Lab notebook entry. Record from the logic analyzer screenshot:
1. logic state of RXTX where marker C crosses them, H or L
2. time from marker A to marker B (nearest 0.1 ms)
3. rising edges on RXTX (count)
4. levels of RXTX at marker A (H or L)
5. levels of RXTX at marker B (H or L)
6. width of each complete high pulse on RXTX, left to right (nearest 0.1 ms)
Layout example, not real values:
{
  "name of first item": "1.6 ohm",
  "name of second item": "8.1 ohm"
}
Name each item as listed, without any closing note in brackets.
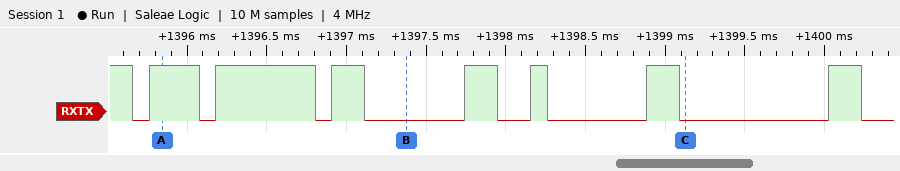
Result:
{
  "logic state of RXTX where marker C crosses them, H or L": "RXTX=L",
  "time from marker A to marker B": "1.5 ms",
  "rising edges on RXTX": "7",
  "levels of RXTX at marker A": "RXTX=H",
  "levels of RXTX at marker B": "RXTX=L",
  "width of each complete high pulse on RXTX, left to right": "0.3 ms, 0.6 ms, 0.2 ms, 0.2 ms, 0.1 ms, 0.2 ms, 0.2 ms"
}
